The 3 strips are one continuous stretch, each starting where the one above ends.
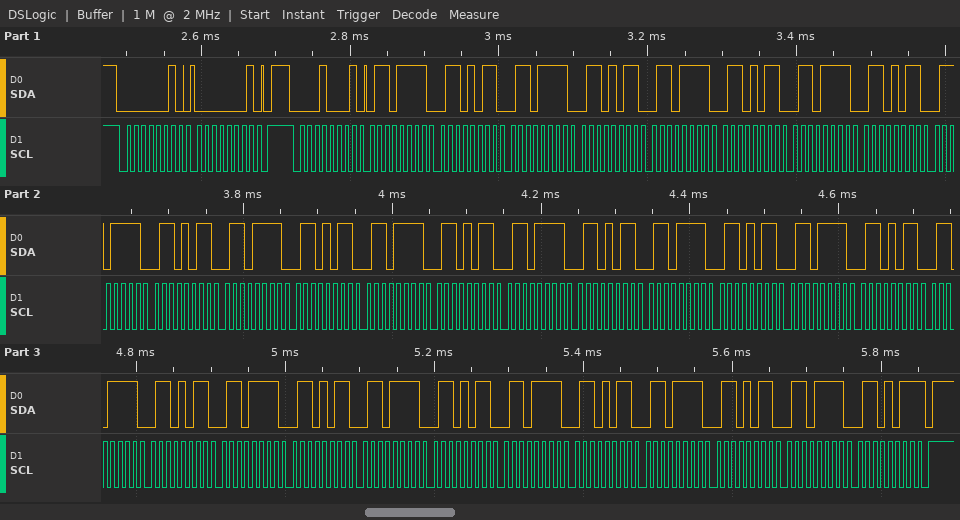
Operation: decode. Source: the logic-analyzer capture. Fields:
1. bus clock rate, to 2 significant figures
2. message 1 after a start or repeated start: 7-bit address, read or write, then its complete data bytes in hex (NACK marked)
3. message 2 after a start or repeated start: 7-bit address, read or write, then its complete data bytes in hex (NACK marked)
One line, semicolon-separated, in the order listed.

100 kHz; 0x01 write: 01; 0x08 read: 6F 6B 6F 6B 6F 6B 6F 6B 6F 6B 6F 6B 6F 6B 6F 6B 6F 6B 6F 6B 6F 6B 6F 6B 6F 6B 6F 6B 6F 6B 6F 6B NACK
